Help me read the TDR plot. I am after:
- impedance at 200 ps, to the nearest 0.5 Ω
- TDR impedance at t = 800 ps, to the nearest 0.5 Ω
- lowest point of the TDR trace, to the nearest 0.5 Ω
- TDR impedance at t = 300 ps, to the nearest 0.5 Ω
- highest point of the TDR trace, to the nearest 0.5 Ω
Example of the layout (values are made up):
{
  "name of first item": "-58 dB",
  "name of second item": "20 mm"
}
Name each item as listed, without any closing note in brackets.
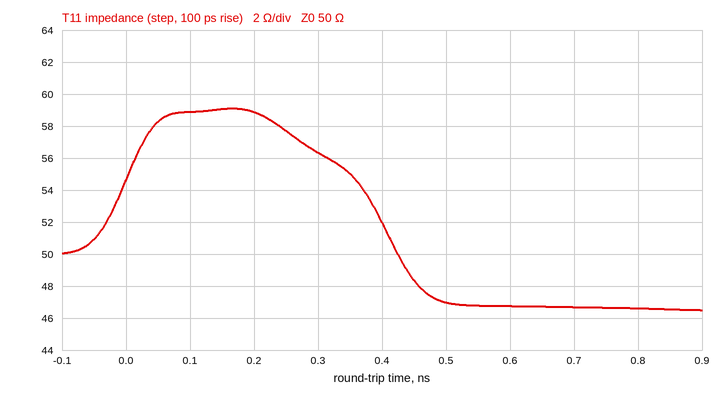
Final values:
{
  "impedance at 200 ps, to the nearest 0.5 Ω": "59.0 Ω",
  "TDR impedance at t = 800 ps, to the nearest 0.5 Ω": "46.5 Ω",
  "lowest point of the TDR trace, to the nearest 0.5 Ω": "46.5 Ω",
  "TDR impedance at t = 300 ps, to the nearest 0.5 Ω": "56.5 Ω",
  "highest point of the TDR trace, to the nearest 0.5 Ω": "59.0 Ω"
}
